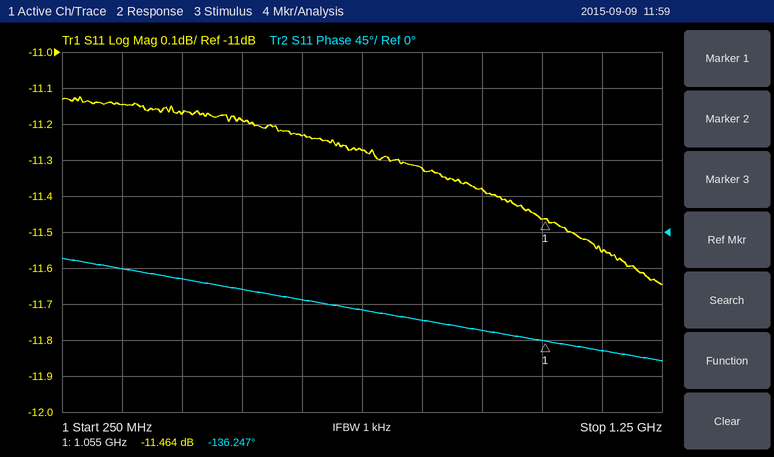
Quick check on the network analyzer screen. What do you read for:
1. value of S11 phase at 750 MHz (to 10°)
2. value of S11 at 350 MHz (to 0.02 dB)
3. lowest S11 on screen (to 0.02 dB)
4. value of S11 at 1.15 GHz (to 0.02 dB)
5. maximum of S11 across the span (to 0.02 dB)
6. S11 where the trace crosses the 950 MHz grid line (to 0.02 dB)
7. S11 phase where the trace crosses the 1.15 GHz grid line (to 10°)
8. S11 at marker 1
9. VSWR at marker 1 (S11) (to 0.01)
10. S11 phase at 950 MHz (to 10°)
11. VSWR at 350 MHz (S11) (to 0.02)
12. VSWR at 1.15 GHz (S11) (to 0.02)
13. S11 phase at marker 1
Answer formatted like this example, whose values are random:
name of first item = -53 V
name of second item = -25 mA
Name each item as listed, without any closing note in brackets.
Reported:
value of S11 phase at 750 MHz = -100°
value of S11 at 350 MHz = -11.14 dB
lowest S11 on screen = -11.64 dB
value of S11 at 1.15 GHz = -11.56 dB
maximum of S11 across the span = -11.12 dB
S11 where the trace crosses the 950 MHz grid line = -11.38 dB
S11 phase where the trace crosses the 1.15 GHz grid line = -150°
S11 at marker 1 = -11.464 dB
VSWR at marker 1 (S11) = 1.73
S11 phase at 950 MHz = -120°
VSWR at 350 MHz (S11) = 1.76
VSWR at 1.15 GHz (S11) = 1.72
S11 phase at marker 1 = -136.247°
